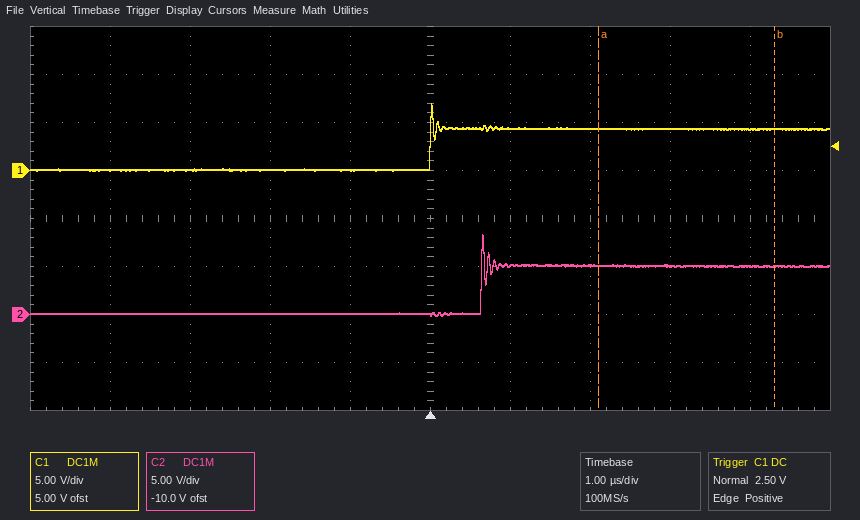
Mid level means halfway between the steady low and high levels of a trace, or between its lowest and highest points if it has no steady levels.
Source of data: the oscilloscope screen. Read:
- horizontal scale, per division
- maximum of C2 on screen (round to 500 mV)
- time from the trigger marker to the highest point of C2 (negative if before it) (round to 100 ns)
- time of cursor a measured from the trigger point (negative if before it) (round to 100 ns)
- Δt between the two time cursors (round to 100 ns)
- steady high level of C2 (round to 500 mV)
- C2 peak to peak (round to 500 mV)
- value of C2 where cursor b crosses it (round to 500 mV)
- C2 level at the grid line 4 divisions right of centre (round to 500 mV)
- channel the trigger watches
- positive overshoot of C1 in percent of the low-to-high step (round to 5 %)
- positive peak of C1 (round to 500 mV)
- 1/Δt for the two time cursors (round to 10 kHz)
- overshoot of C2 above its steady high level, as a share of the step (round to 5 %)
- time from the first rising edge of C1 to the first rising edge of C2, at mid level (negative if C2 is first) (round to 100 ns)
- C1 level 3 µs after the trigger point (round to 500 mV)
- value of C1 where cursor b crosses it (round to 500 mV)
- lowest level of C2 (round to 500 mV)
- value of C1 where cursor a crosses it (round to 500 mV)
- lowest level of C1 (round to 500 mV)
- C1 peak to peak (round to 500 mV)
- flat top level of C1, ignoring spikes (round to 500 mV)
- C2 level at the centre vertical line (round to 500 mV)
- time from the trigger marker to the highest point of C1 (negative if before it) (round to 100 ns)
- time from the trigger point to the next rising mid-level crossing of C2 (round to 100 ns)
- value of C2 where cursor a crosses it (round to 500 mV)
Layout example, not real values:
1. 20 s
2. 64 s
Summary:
1. 1 µs
2. 8.5 V
3. +700 ns
4. +2.1 µs
5. 2.2 µs
6. 5.0 V
7. 8.5 V
8. 5.0 V
9. 5.0 V
10. C1
11. 60 %
12. 7.0 V
13. 450 kHz
14. 65 %
15. +600 ns
16. 4.5 V
17. 4.5 V
18. 0.0 V
19. 4.5 V
20. 0.0 V
21. 7.0 V
22. 4.5 V
23. 0.0 V
24. 0.0 µs
25. 600 ns
26. 5.0 V
